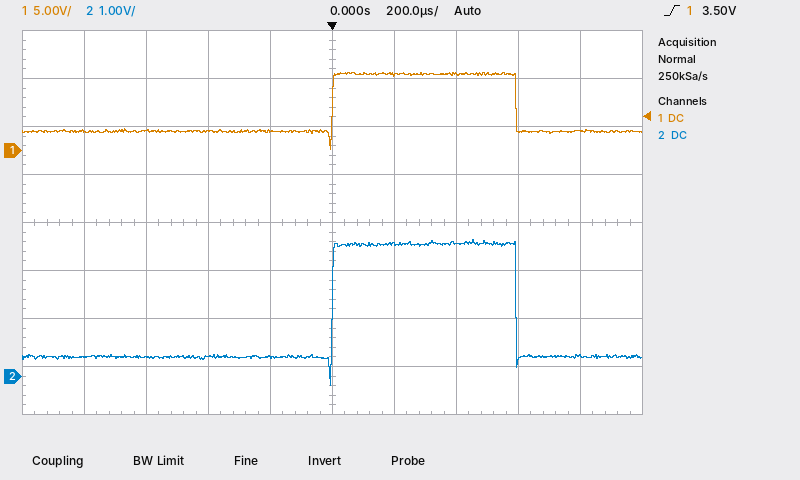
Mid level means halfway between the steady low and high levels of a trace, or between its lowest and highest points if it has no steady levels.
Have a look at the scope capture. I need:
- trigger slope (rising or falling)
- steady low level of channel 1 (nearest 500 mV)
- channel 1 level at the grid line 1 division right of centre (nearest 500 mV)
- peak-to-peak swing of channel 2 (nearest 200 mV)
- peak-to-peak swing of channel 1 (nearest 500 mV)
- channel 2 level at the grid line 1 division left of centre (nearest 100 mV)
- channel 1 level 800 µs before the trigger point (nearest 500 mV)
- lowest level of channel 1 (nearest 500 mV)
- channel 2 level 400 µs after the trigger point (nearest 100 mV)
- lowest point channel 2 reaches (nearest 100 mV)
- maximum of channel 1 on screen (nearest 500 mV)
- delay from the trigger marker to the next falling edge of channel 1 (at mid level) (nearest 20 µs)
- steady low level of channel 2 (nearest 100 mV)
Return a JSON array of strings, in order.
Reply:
["rising", "2.0 V", "8.0 V", "3.0 V", "8.0 V", "400 mV", "2.0 V", "0.0 V", "2.8 V", "-200 mV", "8.0 V", "600 µs", "400 mV"]
